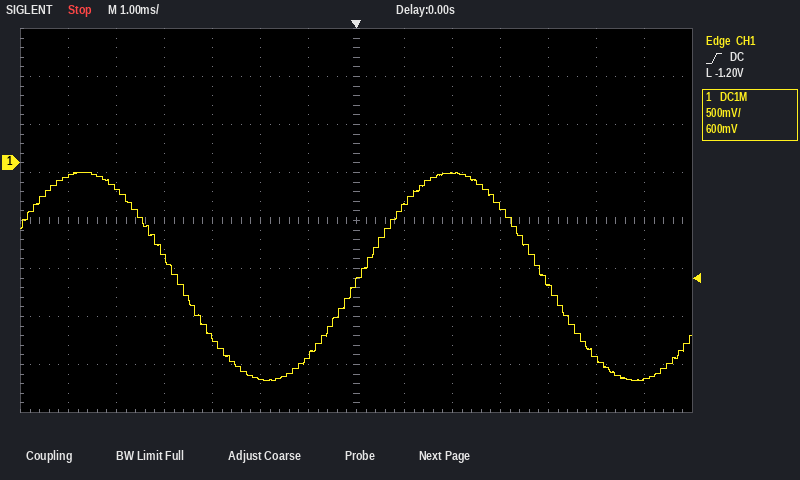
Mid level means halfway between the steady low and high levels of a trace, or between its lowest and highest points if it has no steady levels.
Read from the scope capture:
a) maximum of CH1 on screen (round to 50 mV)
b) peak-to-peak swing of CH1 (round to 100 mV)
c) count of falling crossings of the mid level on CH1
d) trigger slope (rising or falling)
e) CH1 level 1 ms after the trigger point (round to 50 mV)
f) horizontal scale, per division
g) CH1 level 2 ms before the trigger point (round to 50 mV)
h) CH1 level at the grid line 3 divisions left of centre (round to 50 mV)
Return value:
-100 mV
2.20 V
2
rising
-450 mV
1 ms
-2.25 V
-1.80 V
